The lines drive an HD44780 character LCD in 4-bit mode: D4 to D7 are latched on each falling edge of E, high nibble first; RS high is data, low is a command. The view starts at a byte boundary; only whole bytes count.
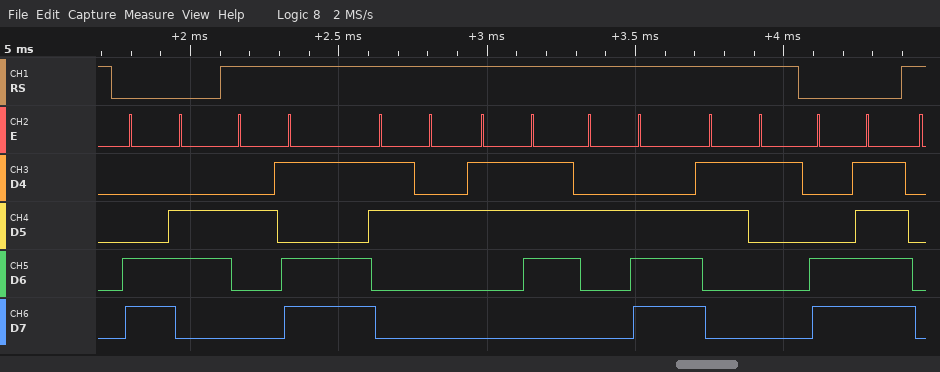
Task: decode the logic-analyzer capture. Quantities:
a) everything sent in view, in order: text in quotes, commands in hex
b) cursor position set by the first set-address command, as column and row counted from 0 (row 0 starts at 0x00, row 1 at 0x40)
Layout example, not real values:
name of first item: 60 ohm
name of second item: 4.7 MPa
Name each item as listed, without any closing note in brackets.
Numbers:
everything sent in view, in order: text in quotes, commands in hex: 0xC6 "-27.1" 0xCF
cursor position set by the first set-address command, as column and row counted from 0: column 6, row 1
